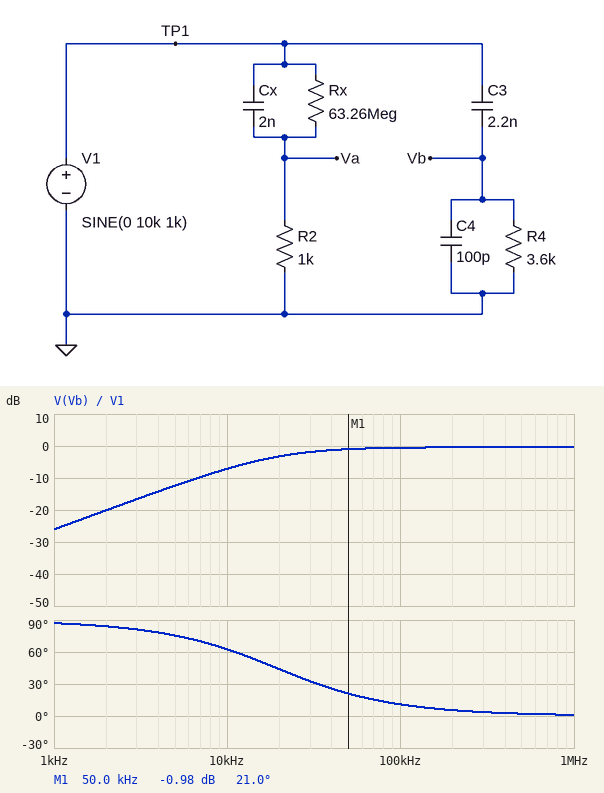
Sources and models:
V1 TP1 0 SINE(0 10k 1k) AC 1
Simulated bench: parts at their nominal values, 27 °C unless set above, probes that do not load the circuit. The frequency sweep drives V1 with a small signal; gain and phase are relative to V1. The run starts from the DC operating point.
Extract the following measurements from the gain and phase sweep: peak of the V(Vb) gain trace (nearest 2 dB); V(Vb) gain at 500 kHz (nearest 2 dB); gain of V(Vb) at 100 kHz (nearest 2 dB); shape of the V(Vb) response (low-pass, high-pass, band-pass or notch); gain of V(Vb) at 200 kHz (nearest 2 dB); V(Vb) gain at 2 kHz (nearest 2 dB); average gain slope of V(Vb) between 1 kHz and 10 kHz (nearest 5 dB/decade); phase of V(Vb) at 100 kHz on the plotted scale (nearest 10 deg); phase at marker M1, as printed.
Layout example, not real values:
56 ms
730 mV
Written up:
0 dB
0 dB
0 dB
high-pass
0 dB
-20 dB
20 dB/decade
10 deg
21.0 deg
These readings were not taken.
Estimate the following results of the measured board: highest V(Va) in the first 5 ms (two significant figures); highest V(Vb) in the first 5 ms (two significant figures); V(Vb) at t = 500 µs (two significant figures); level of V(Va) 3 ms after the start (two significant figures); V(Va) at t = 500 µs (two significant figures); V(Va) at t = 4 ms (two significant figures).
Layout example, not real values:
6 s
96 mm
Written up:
130 V
500 V
-500 V
130 V
-130 V
130 V
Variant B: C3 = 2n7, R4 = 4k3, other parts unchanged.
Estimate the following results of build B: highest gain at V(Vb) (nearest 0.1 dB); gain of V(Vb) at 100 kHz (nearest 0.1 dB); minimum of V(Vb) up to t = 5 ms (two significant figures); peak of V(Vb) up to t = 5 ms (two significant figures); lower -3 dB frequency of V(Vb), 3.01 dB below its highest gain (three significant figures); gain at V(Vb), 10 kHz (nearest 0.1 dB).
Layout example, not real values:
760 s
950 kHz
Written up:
-0.3 dB
-0.4 dB
-730 V
730 V
13.2 kHz
-4.7 dB
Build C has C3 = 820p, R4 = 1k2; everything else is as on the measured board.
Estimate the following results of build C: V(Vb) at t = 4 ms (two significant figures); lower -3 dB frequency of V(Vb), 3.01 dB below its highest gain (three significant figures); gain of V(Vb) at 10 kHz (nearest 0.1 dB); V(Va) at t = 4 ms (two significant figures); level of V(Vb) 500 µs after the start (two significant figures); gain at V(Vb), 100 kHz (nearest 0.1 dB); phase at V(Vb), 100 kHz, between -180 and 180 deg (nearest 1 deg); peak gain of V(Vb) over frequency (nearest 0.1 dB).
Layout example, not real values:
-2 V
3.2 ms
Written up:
62 V
144 kHz
-24.2 dB
130 V
-62 V
-5.9 dB
55 deg
-1.0 dB
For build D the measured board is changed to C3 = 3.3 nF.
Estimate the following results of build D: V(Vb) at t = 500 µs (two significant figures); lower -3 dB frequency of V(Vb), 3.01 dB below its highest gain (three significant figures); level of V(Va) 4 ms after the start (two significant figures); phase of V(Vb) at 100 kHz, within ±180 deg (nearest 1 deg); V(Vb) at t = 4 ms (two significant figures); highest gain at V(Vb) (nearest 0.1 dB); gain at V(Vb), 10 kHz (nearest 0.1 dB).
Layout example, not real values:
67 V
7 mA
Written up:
-740 V
13.0 kHz
130 V
7 deg
740 V
-0.3 dB
-4.6 dB
